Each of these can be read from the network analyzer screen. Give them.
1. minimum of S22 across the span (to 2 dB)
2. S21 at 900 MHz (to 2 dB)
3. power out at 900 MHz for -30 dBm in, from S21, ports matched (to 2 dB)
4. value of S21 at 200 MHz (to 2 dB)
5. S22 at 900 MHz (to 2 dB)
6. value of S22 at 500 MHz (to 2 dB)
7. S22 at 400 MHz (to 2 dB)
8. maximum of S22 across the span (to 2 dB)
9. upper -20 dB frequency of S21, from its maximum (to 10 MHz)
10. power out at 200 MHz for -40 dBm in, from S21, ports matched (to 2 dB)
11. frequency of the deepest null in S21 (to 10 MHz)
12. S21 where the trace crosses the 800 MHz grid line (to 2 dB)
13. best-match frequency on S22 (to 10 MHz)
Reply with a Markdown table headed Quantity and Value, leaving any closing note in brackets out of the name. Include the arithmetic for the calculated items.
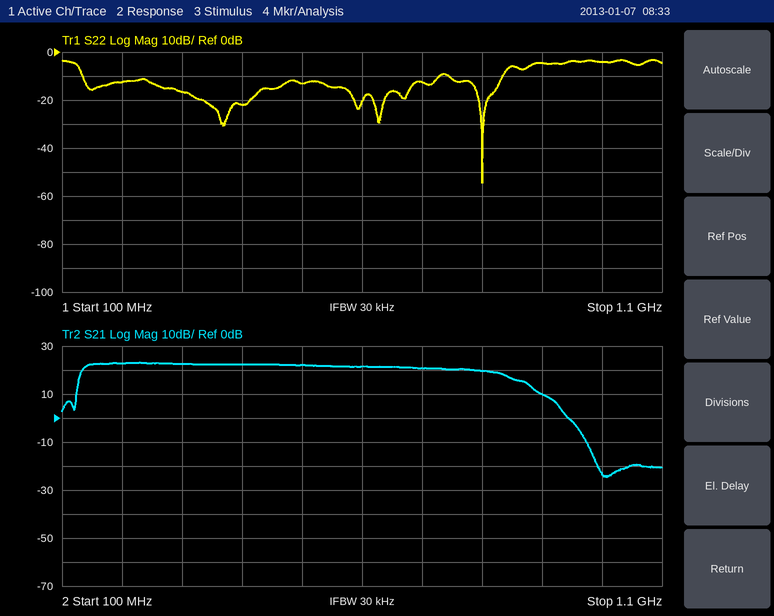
| Quantity | Value |
|---|---|
| minimum of S22 across the span | -54 dB |
| S21 at 900 MHz | 10 dB |
| power out at 900 MHz for -30 dBm in, from S21, ports matched | -30 dBm + (10 dB) = -20 dBm |
| value of S21 at 200 MHz | 22 dB |
| S22 at 900 MHz | -4 dB |
| value of S22 at 500 MHz | -14 dB |
| S22 at 400 MHz | -22 dB |
| maximum of S22 across the span | -4 dB |
| upper -20 dB frequency of S21, from its maximum | 930 MHz |
| power out at 200 MHz for -40 dBm in, from S21, ports matched | -40 dBm + (22 dB) = -18 dBm |
| frequency of the deepest null in S21 | 1.01 GHz |
| S21 where the trace crosses the 800 MHz grid line | 20 dB |
| best-match frequency on S22 | 800 MHz |
